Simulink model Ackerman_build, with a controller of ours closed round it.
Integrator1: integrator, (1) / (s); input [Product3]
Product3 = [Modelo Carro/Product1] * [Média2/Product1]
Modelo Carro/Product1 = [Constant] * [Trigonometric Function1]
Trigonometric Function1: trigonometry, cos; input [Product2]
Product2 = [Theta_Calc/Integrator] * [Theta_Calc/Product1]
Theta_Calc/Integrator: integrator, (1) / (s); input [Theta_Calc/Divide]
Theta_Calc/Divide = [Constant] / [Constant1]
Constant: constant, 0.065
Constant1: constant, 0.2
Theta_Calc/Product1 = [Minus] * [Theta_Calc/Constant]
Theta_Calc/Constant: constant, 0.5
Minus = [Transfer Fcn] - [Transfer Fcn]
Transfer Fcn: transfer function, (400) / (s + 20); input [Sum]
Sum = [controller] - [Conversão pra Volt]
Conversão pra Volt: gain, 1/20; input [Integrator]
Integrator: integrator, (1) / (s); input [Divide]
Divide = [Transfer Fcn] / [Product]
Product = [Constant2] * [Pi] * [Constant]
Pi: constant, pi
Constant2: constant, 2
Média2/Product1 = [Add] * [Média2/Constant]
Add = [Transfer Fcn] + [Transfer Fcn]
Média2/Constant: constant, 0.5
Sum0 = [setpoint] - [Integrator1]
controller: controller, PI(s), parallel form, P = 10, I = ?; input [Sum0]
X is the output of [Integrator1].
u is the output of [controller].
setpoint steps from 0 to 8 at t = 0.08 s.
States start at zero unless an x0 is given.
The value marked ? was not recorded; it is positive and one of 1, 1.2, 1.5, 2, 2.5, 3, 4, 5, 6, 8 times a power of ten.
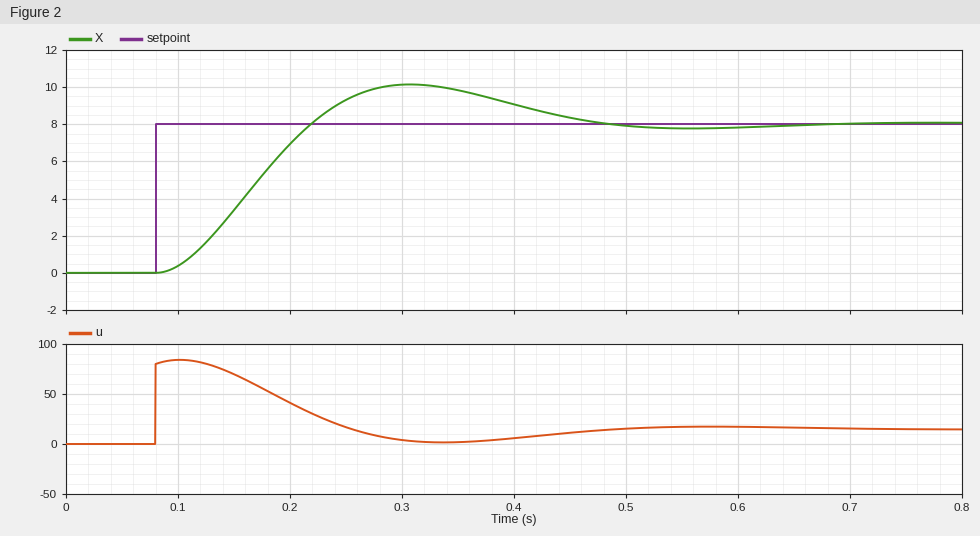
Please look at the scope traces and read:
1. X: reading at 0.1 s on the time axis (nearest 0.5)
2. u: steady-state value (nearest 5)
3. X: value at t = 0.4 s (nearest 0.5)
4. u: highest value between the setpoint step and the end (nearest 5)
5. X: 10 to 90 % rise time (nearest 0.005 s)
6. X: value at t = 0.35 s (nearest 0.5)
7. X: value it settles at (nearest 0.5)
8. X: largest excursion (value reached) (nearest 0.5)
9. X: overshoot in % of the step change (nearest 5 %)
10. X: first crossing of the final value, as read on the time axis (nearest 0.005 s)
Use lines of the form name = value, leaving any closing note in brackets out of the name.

X: reading at 0.1 s on the time axis = 0.5
u: steady-state value = 15
X: value at t = 0.4 s = 9.0
u: highest value between the setpoint step and the end = 85
X: 10 to 90 % rise time = 0.095 s
X: value at t = 0.35 s = 10.0
X: value it settles at = 8.0
X: largest excursion (value reached) = 10.0
X: overshoot in % of the step change = 25 %
X: first crossing of the final value, as read on the time axis = 0.220 s
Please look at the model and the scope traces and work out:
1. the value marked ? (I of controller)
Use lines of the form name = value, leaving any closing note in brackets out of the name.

the value marked ? = 50
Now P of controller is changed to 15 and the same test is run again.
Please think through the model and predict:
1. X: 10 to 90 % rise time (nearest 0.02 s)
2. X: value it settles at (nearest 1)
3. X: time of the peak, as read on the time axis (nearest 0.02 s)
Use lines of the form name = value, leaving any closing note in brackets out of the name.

X: 10 to 90 % rise time = 0.08 s
X: value it settles at = 8
X: time of the peak, as read on the time axis = 0.26 s
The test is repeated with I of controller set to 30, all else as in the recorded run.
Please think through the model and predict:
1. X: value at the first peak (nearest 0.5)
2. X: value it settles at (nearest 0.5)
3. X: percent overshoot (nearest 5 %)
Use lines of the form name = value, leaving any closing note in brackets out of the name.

X: value at the first peak = 9.0
X: value it settles at = 8.0
X: percent overshoot = 15 %
